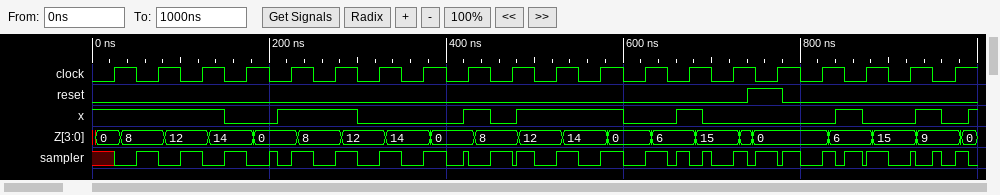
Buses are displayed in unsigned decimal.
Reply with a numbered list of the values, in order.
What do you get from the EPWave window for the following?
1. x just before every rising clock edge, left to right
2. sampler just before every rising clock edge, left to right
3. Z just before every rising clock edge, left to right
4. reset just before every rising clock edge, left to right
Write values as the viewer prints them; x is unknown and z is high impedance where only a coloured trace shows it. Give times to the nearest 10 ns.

1. 1 1 1 0 1 1 0 0 1 0 1 1 0 1 0 0 0 0 0 0
2. x 1 1 1 0 0 0 0 1 1 0 0 0 1 0 1 0 0 0 0
3. 0, 8, 12, 14, 0, 8, 12, 14, 0, 8, 12, 14, 0, 6, 15, 0, 0, 6, 15, 9
4. 0 0 0 0 0 0 0 0 0 0 0 0 0 0 0 1 0 0 0 0
